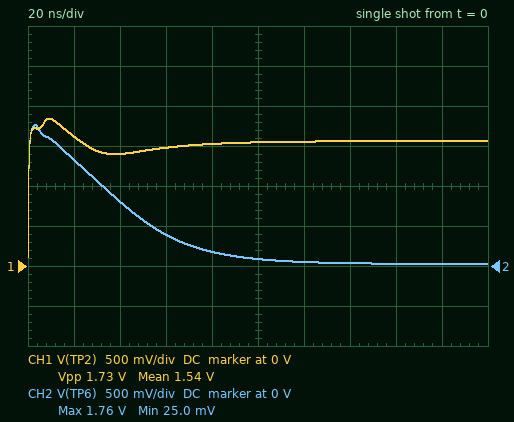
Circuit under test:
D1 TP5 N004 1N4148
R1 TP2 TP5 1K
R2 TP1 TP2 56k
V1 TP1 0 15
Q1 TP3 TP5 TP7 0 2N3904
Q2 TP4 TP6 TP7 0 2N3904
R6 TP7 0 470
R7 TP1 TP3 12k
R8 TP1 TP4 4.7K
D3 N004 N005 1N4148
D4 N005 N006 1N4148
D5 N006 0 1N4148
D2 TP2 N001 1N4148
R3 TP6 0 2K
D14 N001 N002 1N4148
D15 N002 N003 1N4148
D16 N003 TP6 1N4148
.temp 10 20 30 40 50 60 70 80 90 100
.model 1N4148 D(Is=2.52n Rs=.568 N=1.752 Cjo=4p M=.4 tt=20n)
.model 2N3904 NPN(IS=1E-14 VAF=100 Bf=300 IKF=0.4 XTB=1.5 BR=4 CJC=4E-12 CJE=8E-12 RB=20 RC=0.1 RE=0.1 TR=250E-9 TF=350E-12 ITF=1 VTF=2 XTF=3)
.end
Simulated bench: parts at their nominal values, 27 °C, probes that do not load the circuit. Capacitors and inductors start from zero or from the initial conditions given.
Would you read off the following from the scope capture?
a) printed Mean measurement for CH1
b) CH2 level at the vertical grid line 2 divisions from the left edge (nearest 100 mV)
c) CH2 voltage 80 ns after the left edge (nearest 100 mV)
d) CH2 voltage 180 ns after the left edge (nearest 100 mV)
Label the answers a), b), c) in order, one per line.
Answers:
a) 1.54 V
b) 800 mV
c) 200 mV
d) 0 V
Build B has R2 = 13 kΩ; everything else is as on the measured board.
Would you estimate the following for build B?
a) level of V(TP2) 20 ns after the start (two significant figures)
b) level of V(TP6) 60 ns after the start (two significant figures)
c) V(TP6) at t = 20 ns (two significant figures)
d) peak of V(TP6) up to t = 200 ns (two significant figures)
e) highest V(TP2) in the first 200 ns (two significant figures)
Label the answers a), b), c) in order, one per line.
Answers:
a) 2.6 V
b) 520 mV
c) 1.6 V
d) 1.9 V
e) 2.8 V
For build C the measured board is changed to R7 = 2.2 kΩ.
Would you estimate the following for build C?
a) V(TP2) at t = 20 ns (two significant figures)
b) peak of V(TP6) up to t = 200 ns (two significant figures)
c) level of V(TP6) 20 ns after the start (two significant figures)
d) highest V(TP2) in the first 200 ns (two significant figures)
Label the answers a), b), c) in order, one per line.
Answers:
a) 2.2 V
b) 2.1 V
c) 1.8 V
d) 2.4 V
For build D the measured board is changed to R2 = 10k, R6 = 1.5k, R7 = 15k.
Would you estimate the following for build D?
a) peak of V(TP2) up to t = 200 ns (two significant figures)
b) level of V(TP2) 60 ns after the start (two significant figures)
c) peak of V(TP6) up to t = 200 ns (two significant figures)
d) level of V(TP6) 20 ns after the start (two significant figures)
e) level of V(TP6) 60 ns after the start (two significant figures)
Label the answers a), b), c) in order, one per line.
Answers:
a) 3.3 V
b) 3.0 V
c) 2.6 V
d) 1.9 V
e) 910 mV
